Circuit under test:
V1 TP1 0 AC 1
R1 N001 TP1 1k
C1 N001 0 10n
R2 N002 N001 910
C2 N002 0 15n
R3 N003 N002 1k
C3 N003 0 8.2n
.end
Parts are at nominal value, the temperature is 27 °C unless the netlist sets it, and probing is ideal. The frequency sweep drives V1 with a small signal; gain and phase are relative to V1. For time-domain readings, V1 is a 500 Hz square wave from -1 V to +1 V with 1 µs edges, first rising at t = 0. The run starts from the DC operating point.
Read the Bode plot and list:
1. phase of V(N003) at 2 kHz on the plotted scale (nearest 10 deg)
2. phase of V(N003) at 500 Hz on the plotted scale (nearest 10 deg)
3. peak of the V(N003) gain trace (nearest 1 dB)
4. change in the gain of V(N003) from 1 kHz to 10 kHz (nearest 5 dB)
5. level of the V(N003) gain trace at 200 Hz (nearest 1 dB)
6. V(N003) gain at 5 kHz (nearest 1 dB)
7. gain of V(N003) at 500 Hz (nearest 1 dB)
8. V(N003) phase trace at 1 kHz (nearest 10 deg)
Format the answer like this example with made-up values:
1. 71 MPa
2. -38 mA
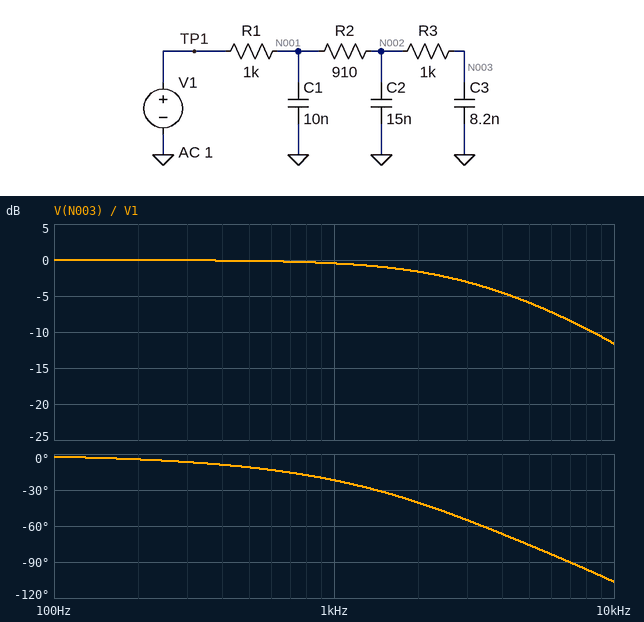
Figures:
1. -40 deg
2. -10 deg
3. 0 dB
4. -10 dB
5. 0 dB
6. -6 dB
7. 0 dB
8. -20 deg
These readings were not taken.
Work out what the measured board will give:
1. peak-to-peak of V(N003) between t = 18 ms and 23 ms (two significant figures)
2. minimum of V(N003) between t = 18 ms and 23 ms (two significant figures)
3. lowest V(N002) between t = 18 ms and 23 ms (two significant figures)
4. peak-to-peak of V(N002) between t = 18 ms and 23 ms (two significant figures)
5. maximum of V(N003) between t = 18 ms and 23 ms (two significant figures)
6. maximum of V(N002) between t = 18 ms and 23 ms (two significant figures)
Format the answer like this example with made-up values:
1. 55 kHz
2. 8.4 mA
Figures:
1. 2.0 V
2. -1.0 V
3. -1.0 V
4. 2.0 V
5. 1.0 V
6. 1.0 V
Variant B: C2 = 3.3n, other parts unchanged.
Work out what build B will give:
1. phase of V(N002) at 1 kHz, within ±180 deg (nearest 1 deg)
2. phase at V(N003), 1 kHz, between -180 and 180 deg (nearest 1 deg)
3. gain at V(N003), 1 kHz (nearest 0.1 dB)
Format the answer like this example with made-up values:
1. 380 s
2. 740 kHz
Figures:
1. -11 deg
2. -14 deg
3. -0.2 dB
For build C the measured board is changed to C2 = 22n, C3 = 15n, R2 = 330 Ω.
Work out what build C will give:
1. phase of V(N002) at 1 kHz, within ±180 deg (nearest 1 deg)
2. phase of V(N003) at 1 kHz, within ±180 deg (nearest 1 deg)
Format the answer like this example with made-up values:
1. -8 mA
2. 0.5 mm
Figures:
1. -20 deg
2. -26 deg
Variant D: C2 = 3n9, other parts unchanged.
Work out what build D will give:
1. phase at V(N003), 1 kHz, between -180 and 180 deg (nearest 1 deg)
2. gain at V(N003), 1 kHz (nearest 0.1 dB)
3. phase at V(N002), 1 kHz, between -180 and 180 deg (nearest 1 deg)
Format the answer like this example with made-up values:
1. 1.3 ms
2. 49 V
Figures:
1. -15 deg
2. -0.2 dB
3. -12 deg
